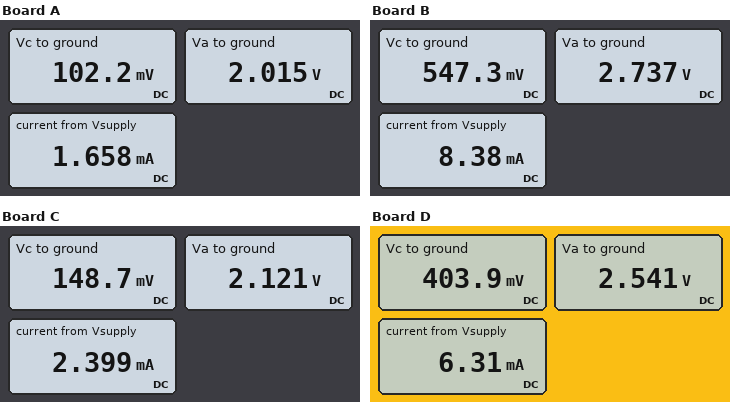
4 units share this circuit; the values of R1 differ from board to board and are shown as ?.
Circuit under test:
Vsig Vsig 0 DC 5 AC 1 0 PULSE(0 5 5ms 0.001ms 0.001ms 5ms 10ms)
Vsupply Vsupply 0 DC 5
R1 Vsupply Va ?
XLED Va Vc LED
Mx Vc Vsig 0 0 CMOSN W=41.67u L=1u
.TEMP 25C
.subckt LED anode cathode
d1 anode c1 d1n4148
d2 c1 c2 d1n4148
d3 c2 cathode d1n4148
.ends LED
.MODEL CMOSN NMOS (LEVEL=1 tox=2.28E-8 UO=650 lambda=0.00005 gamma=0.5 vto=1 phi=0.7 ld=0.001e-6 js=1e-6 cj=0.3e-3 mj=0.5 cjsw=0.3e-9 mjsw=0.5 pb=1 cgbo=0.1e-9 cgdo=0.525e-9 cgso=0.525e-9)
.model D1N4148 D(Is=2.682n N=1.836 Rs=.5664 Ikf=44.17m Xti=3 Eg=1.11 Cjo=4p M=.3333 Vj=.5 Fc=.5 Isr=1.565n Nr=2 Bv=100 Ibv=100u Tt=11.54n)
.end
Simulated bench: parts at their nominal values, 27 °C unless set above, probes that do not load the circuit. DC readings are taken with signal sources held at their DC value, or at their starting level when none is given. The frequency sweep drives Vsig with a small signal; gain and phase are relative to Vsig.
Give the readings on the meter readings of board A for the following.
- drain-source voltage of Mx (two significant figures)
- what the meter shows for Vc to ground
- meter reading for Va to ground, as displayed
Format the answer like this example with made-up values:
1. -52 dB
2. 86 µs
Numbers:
1. 100 mV
2. 102.2 mV
3. 2.015 V
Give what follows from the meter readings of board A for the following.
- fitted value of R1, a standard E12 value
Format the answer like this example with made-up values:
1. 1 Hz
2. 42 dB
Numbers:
1. 1.8 kΩ
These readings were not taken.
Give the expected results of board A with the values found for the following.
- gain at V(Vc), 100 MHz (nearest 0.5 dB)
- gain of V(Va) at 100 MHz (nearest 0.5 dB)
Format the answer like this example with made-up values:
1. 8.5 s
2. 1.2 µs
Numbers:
1. -32.0 dB
2. -32.0 dB
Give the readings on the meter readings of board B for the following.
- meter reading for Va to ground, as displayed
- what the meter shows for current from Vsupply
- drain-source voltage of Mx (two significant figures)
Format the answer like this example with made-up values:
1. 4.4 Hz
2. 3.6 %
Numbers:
1. 2.737 V
2. 8.38 mA
3. 550 mV
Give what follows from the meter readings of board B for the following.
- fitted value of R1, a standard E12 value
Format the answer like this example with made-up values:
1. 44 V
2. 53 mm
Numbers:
1. 270 Ω
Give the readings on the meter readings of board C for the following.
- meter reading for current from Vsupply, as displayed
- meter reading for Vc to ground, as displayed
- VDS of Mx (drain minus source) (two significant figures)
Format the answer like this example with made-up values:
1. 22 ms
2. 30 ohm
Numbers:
1. 2.399 mA
2. 148.7 mV
3. 150 mV
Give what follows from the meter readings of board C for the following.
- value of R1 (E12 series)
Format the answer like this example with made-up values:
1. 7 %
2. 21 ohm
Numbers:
1. 1.2 kΩ
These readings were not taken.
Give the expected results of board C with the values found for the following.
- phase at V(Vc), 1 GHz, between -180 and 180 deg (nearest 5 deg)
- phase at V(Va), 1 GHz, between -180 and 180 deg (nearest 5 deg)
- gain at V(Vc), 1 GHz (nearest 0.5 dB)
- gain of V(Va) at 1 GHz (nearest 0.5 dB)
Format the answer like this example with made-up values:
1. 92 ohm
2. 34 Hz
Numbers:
1. 150 deg
2. 150 deg
3. -27.5 dB
4. -27.5 dB
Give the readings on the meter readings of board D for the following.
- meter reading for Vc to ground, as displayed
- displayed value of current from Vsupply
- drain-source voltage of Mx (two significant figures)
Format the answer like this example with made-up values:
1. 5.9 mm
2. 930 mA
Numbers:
1. 403.9 mV
2. 6.31 mA
3. 400 mV
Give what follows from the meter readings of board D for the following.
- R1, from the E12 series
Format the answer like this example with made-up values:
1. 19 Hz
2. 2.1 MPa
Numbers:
1. 390 Ω
